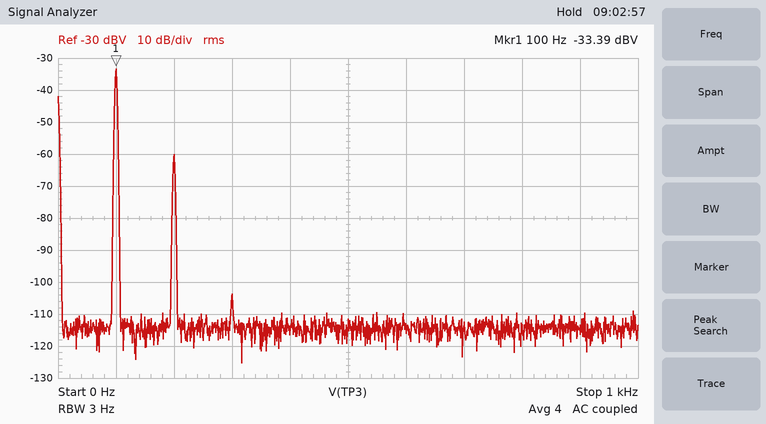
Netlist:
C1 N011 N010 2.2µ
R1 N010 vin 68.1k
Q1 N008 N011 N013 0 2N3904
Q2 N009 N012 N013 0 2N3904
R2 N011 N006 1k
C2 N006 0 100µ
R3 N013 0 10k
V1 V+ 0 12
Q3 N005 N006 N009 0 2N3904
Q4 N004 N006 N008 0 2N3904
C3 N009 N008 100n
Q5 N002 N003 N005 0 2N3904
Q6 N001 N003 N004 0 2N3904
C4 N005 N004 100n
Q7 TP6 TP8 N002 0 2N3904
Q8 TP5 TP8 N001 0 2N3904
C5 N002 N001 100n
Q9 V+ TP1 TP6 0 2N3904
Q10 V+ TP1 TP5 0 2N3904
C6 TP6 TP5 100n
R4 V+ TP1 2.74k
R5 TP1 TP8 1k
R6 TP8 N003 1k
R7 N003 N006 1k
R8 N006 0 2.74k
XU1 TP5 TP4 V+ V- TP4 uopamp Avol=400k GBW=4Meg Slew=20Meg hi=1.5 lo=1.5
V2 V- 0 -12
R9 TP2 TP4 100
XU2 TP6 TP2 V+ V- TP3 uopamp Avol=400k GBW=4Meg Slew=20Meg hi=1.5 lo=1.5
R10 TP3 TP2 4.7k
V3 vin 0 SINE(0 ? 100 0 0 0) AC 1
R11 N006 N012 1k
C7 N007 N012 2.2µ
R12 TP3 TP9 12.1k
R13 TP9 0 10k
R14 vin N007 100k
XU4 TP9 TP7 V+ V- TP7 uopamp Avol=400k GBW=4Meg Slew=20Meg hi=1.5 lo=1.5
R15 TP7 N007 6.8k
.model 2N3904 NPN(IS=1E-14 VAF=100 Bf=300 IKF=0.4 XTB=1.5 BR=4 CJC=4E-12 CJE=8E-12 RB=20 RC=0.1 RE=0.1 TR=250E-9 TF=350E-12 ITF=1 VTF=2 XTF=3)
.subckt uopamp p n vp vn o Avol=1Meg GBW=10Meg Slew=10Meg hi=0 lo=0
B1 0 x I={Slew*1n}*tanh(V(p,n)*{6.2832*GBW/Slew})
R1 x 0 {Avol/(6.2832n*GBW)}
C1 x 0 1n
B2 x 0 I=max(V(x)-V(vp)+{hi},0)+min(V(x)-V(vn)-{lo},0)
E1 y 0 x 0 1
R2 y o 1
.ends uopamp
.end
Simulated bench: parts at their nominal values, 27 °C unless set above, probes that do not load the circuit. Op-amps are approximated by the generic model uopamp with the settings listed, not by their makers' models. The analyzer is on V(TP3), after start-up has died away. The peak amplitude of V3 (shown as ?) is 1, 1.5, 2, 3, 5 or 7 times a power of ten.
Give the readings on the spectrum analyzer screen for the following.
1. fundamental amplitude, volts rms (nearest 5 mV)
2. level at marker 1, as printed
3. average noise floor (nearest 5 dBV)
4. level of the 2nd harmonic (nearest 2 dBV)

20 mV
-33.39 dBV
-115 dBV
-60 dBV
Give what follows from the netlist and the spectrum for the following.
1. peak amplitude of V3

700 mV
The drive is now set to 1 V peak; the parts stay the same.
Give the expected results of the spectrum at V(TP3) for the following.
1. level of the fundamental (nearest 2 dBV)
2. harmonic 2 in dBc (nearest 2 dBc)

-30 dBV
-24 dBc
